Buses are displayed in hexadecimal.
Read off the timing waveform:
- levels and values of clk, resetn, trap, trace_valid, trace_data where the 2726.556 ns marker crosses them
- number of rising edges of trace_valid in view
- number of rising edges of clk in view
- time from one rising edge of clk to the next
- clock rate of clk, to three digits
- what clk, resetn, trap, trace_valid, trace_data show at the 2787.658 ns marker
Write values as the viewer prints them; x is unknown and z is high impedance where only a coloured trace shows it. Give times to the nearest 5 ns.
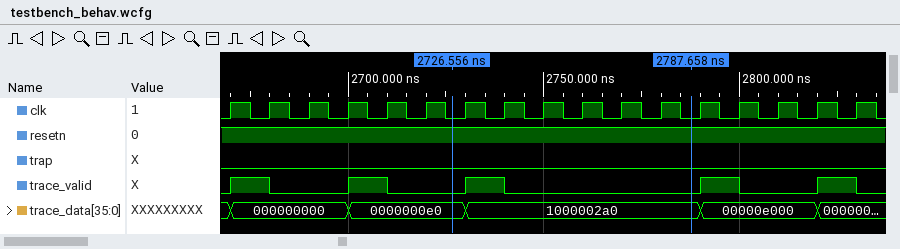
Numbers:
clk=0, resetn=1, trap=0, trace_valid=0, trace_data=0000000e0
5
17
10 ns
100 MHz
clk=0, resetn=1, trap=0, trace_valid=0, trace_data=1000002a0
